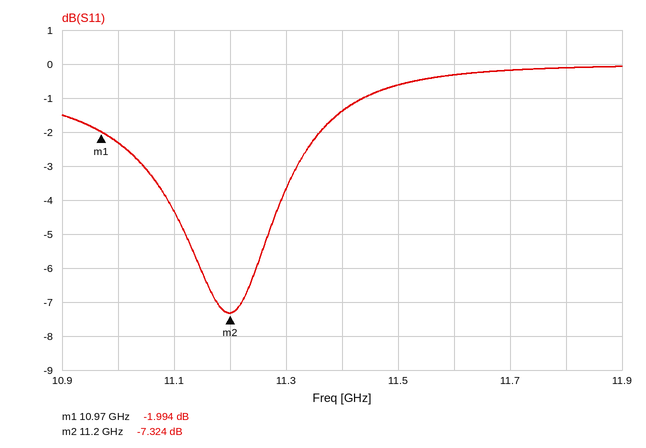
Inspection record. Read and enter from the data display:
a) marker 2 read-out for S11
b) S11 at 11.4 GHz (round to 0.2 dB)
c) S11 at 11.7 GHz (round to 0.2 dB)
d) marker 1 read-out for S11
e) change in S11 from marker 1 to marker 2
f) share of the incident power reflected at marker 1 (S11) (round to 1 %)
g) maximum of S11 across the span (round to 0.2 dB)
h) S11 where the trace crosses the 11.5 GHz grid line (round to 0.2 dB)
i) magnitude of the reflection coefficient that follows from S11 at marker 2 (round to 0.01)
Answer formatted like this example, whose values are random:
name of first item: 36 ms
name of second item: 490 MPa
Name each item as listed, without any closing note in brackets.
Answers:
marker 2 read-out for S11: -7.324 dB
S11 at 11.4 GHz: -1.4 dB
S11 at 11.7 GHz: -0.2 dB
marker 1 read-out for S11: -1.994 dB
change in S11 from marker 1 to marker 2: -5.330 dB
share of the incident power reflected at marker 1 (S11): 63 %
maximum of S11 across the span: 0.0 dB
S11 where the trace crosses the 11.5 GHz grid line: -0.6 dB
magnitude of the reflection coefficient that follows from S11 at marker 2: 0.43
